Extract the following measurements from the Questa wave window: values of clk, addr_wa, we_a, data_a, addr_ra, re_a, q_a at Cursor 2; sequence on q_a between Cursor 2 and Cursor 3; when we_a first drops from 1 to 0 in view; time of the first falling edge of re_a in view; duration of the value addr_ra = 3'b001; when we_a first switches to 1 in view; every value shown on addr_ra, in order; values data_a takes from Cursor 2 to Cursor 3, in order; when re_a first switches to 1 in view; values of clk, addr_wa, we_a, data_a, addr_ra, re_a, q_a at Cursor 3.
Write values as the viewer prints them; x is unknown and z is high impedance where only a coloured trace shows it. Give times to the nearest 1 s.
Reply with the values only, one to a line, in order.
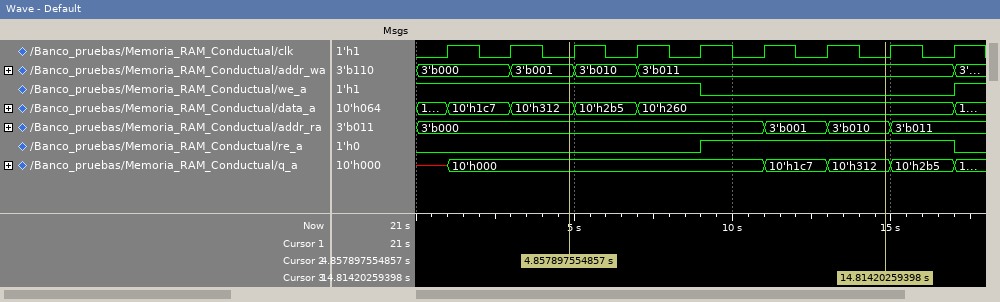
clk=0, addr_wa=3'b001, we_a=1, data_a=10'h312, addr_ra=3'b000, re_a=0, q_a=10'h000
10'h000, 10'h1c7, 10'h312
9 s
17 s
2 s
17 s
3'b000, 3'b001, 3'b010, 3'b011
10'h312, 10'h2b5, 10'h260
9 s
clk=0, addr_wa=3'b011, we_a=0, data_a=10'h260, addr_ra=3'b010, re_a=1, q_a=10'h312
